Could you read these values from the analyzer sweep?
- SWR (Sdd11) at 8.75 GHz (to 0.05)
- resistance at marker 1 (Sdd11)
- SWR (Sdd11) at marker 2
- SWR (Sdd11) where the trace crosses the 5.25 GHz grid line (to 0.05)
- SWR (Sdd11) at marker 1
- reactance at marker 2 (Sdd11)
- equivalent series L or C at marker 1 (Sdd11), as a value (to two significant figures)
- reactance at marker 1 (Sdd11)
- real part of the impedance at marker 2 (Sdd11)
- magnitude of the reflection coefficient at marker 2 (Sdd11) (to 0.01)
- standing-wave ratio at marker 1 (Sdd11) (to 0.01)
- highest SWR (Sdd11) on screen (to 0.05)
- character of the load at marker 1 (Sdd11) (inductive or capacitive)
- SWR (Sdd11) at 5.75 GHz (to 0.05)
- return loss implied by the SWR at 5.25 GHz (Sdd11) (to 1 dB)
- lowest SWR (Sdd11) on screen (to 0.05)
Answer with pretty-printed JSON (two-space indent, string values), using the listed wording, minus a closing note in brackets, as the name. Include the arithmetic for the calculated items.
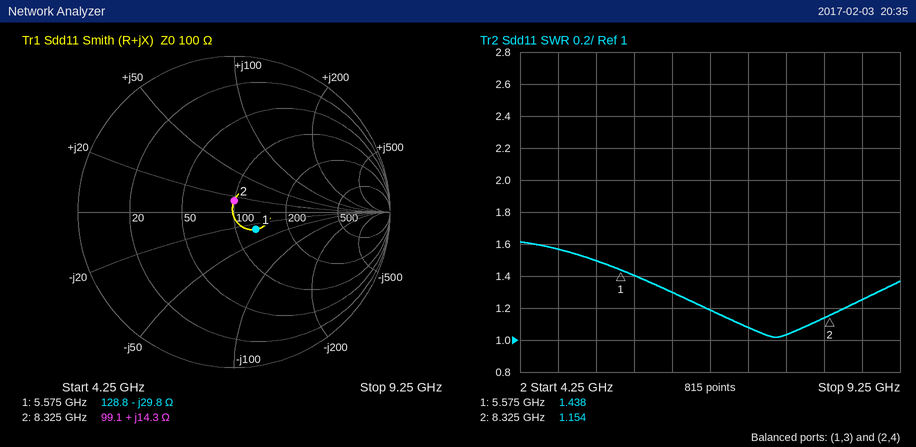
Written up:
{
  "SWR (Sdd11) at 8.75 GHz": "1.25",
  "resistance at marker 1": "128.8 Ω",
  "SWR (Sdd11) at marker 2": "1.154",
  "SWR (Sdd11) where the trace crosses the 5.25 GHz grid line": "1.50",
  "SWR (Sdd11) at marker 1": "1.438",
  "reactance at marker 2": "+14.3 Ω",
  "equivalent series L or C at marker 1 (Sdd11), as a value": "C = 1/(2π × 5.575 GHz × 29.8 Ω) ≈ 958 fF, so 960 fF to two significant figures",
  "reactance at marker 1": "-29.8 Ω",
  "real part of the impedance at marker 2": "99.1 Ω",
  "magnitude of the reflection coefficient at marker 2 (Sdd11)": "0.07",
  "standing-wave ratio at marker 1 (Sdd11)": "1.44",
  "highest SWR (Sdd11) on screen": "1.60",
  "character of the load at marker 1 (Sdd11)": "capacitive",
  "SWR (Sdd11) at 5.75 GHz": "1.40",
  "return loss implied by the SWR at 5.25 GHz (Sdd11)": "−20 log10((1.5 − 1)/(1.5 + 1)) ≈ 14 dB",
  "lowest SWR (Sdd11) on screen": "1.00"
}
